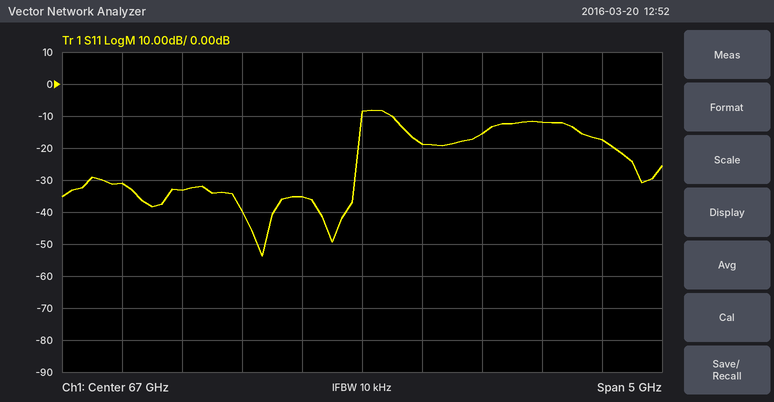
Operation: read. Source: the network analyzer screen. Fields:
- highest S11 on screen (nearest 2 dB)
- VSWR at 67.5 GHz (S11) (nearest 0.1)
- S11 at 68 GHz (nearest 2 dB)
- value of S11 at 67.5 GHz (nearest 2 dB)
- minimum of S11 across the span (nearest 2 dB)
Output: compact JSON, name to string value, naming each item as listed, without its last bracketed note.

{"highest S11 on screen": "-8 dB", "VSWR at 67.5 GHz (S11)": "1.3", "S11 at 68 GHz": "-16 dB", "value of S11 at 67.5 GHz": "-18 dB", "minimum of S11 across the span": "-54 dB"}
